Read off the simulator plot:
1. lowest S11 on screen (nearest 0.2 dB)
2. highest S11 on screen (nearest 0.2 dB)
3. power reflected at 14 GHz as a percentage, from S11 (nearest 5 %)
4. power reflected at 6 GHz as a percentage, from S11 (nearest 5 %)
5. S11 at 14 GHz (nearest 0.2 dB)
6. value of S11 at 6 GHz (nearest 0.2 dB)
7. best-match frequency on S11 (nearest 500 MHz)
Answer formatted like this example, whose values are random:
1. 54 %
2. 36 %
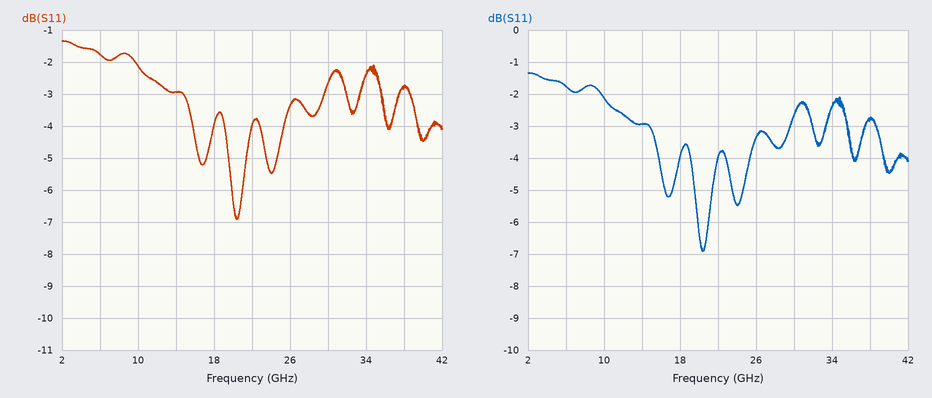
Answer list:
1. -7.0 dB
2. -1.4 dB
3. 50 %
4. 65 %
5. -3.0 dB
6. -1.8 dB
7. 20.5 GHz
